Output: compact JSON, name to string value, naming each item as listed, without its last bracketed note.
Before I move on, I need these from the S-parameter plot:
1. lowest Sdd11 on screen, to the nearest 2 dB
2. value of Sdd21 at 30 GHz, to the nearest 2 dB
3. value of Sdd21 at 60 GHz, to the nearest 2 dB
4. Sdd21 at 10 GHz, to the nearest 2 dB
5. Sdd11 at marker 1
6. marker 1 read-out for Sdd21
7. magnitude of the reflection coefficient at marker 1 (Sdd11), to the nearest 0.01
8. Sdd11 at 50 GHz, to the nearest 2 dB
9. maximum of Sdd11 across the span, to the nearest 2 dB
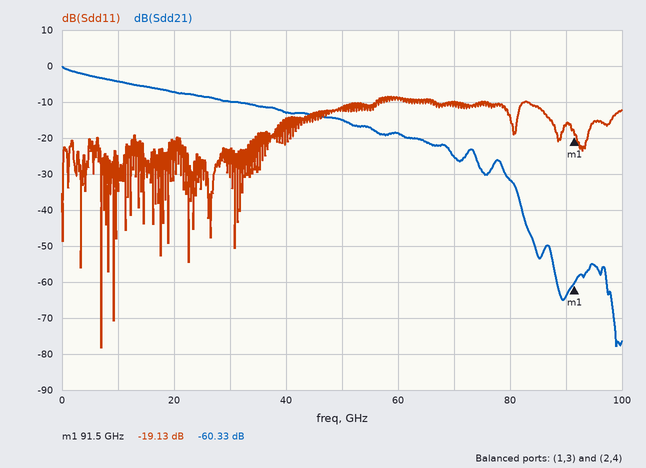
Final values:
{"lowest Sdd11 on screen, to the nearest 2 dB": "-78 dB", "value of Sdd21 at 30 GHz, to the nearest 2 dB": "-10 dB", "value of Sdd21 at 60 GHz, to the nearest 2 dB": "-18 dB", "Sdd21 at 10 GHz, to the nearest 2 dB": "-4 dB", "Sdd11 at marker 1": "-19.13 dB", "marker 1 read-out for Sdd21": "-60.33 dB", "magnitude of the reflection coefficient at marker 1 (Sdd11), to the nearest 0.01": "0.11", "Sdd11 at 50 GHz, to the nearest 2 dB": "-12 dB", "maximum of Sdd11 across the span, to the nearest 2 dB": "-8 dB"}
